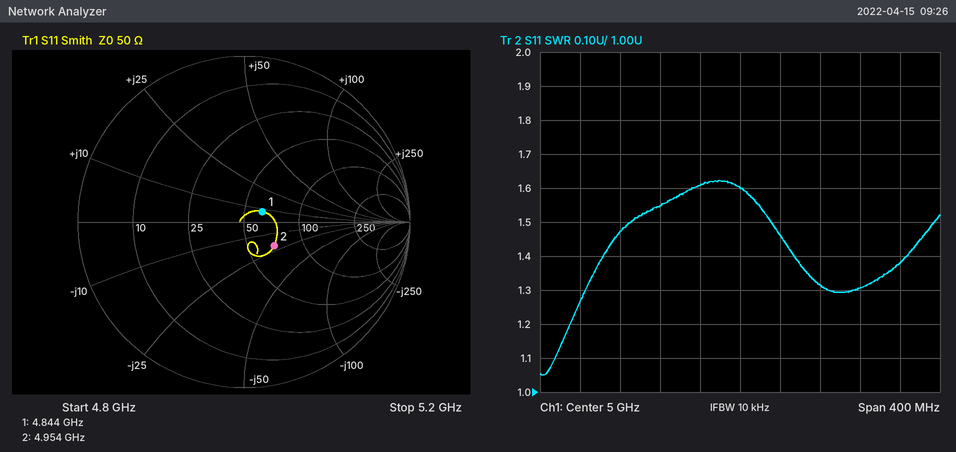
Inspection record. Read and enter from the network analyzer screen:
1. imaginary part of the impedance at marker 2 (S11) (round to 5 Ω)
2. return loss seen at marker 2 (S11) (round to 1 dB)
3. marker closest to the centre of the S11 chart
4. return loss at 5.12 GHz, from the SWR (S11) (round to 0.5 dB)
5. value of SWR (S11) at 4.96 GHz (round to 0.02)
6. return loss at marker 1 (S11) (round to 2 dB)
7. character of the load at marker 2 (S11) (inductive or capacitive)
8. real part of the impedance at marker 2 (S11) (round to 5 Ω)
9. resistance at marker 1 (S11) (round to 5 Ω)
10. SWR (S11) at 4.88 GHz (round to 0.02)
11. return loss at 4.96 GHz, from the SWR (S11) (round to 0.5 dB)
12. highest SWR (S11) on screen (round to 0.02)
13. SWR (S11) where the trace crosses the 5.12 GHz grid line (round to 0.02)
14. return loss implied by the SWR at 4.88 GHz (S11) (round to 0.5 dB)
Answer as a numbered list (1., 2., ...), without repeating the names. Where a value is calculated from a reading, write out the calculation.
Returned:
1. -20 Ω
2. 13 dB
3. marker 1
4. −20 log10((1.3 − 1)/(1.3 + 1)) ≈ 17.7 dB, so 17.5 dB to the nearest 0.5 dB
5. 1.60
6. 18 dB
7. capacitive
8. 70 Ω
9. 60 Ω
10. 1.48
11. −20 log10((1.6 − 1)/(1.6 + 1)) ≈ 12.7 dB, so 12.5 dB to the nearest 0.5 dB
12. 1.62
13. 1.30
14. −20 log10((1.48 − 1)/(1.48 + 1)) ≈ 14.3 dB, so 14.5 dB to the nearest 0.5 dB
